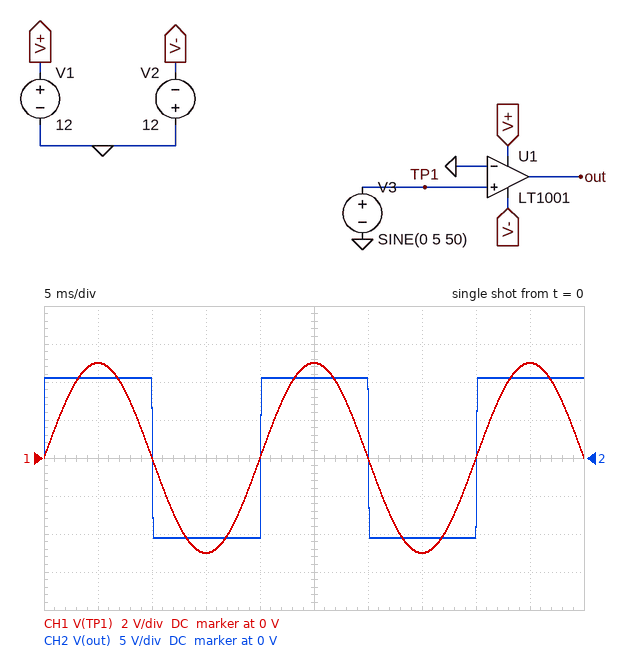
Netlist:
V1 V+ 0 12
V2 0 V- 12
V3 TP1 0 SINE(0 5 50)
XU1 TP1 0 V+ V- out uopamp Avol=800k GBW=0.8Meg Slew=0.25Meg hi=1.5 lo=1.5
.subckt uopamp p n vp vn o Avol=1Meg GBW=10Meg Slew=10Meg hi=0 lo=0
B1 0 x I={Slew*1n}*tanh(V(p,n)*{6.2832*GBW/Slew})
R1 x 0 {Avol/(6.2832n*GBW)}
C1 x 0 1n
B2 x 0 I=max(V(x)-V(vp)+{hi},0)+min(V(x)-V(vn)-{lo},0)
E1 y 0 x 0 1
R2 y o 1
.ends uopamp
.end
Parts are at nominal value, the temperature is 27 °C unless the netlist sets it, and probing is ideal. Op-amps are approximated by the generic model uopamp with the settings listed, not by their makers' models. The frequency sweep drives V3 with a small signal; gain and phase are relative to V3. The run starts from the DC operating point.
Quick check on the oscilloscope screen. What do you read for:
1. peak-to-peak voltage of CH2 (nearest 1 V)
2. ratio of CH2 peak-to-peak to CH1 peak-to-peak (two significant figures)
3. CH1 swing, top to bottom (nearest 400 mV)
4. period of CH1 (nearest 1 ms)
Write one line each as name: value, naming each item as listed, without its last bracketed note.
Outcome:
peak-to-peak voltage of CH2: 21 V
ratio of CH2 peak-to-peak to CH1 peak-to-peak: 2.1
CH1 swing, top to bottom: 10.0 V
period of CH1: 20 ms
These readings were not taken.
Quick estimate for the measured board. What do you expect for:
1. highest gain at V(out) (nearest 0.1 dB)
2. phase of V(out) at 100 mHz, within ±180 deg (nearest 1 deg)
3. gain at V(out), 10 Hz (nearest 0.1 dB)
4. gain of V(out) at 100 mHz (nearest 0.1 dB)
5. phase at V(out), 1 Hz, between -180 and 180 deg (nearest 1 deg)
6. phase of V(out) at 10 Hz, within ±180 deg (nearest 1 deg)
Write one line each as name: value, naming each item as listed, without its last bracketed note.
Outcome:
highest gain at V(out): 118.1 dB
phase of V(out) at 100 mHz, within ±180 deg: -6 deg
gain at V(out), 10 Hz: 98.0 dB
gain of V(out) at 100 mHz: 118.0 dB
phase at V(out), 1 Hz, between -180 and 180 deg: -45 deg
phase of V(out) at 10 Hz, within ±180 deg: -84 deg
